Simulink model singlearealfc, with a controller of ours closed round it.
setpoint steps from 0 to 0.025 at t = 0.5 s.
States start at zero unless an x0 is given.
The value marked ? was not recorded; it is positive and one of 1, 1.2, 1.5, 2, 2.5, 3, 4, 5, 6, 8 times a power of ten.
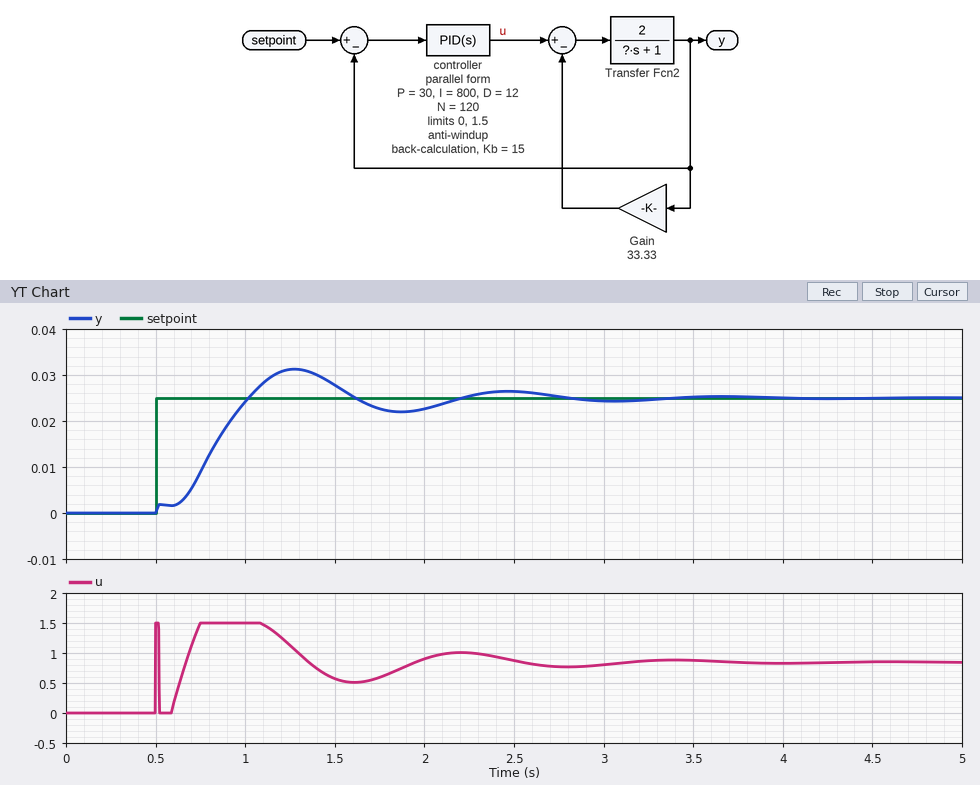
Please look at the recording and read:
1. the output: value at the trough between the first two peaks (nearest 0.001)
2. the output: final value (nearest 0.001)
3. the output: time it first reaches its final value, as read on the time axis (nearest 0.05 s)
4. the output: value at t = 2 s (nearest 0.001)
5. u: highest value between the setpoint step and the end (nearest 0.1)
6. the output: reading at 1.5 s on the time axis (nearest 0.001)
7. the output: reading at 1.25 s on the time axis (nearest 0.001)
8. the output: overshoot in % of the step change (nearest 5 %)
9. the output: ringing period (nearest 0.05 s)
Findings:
0.022
0.025
1.00 s
0.023
1.5
0.028
0.031
25 %
1.20 s
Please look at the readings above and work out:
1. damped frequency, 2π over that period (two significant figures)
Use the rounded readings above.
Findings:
5.2 rad/s
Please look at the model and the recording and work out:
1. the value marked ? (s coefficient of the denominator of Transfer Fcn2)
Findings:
30
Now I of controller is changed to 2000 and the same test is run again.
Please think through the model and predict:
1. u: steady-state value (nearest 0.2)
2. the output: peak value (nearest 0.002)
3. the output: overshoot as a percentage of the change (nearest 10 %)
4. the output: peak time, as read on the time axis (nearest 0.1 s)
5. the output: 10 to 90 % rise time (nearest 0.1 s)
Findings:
0.8
0.030
20 %
1.1 s
0.3 s
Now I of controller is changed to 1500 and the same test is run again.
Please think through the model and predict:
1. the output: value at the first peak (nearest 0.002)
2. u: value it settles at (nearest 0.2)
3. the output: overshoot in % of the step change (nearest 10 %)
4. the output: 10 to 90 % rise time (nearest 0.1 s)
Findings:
0.030
0.8
20 %
0.3 s
